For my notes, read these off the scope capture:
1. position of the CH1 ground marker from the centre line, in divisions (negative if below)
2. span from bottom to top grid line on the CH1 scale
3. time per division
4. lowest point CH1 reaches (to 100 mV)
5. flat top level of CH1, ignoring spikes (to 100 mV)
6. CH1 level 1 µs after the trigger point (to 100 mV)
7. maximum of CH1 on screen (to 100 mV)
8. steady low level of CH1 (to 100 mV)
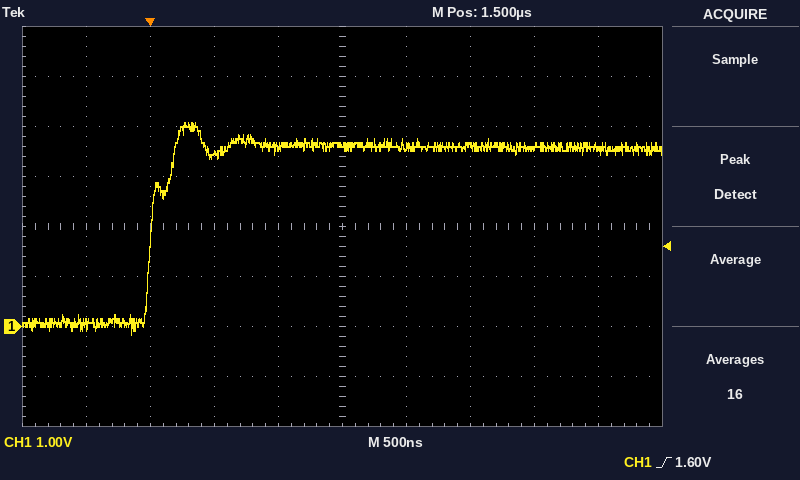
-2.0 div
8 V
500 ns
-200 mV
3.6 V
3.6 V
4.1 V
100 mV
